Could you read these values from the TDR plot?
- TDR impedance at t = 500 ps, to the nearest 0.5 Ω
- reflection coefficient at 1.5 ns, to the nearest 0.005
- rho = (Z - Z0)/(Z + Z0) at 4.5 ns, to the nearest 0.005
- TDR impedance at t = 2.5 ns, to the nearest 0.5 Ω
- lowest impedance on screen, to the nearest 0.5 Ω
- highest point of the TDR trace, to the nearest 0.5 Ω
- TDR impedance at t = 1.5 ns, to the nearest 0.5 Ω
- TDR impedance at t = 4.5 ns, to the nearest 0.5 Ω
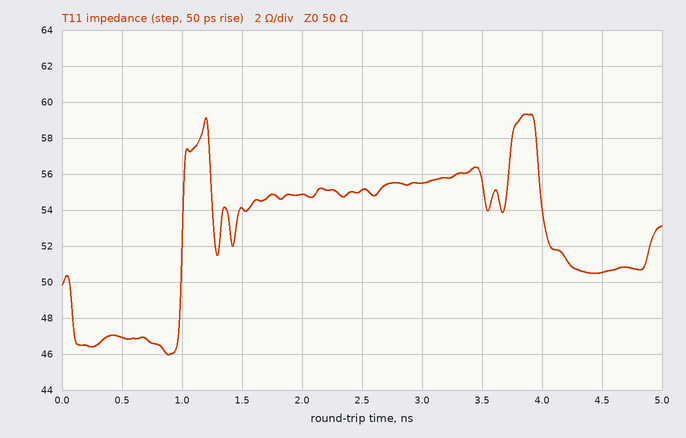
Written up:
47.0 Ω
+0.040
+0.005
55.0 Ω
46.0 Ω
59.5 Ω
54.0 Ω
50.5 Ω
